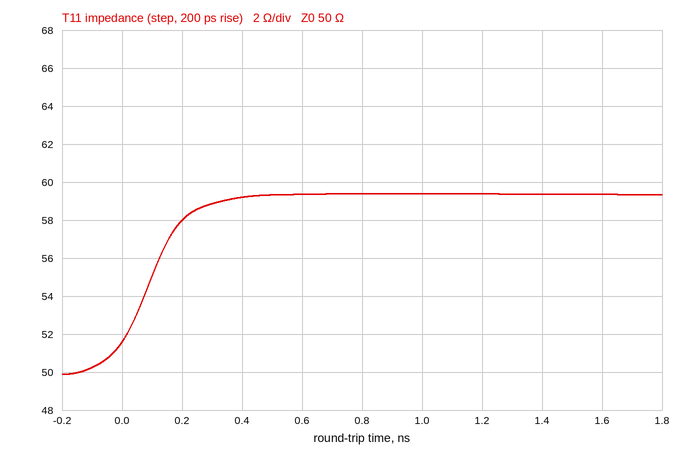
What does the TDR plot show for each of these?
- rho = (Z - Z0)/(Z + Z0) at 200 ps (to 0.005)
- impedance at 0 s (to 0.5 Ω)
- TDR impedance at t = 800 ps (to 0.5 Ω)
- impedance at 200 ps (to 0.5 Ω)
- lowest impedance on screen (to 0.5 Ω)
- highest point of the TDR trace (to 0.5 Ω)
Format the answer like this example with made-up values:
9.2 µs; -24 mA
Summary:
+0.075; 51.5 Ω; 59.5 Ω; 58.0 Ω; 50.0 Ω; 59.5 Ω
